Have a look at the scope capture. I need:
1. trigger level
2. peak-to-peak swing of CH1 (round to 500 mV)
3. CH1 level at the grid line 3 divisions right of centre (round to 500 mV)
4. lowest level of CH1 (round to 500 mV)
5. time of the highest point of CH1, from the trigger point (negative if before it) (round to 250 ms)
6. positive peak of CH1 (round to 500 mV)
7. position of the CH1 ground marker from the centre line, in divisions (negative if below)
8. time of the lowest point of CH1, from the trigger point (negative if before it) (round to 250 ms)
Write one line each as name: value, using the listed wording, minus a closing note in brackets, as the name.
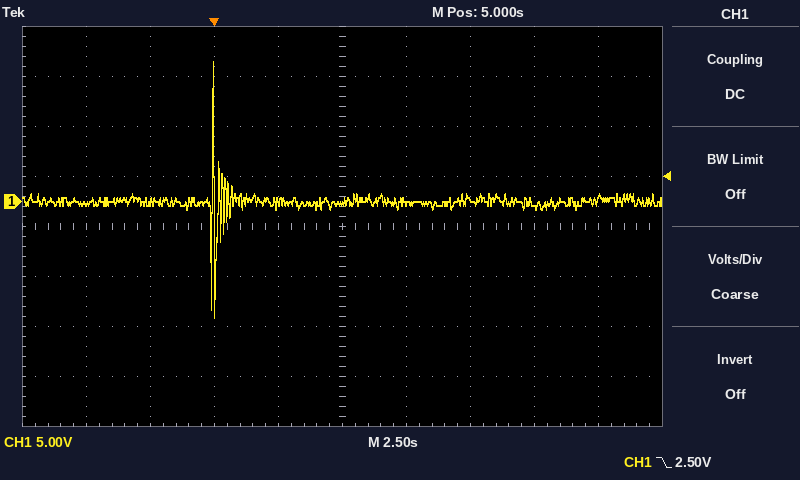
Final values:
trigger level: 2.50 V
peak-to-peak swing of CH1: 25.5 V
CH1 level at the grid line 3 divisions right of centre: -500 mV
lowest level of CH1: -11.5 V
time of the highest point of CH1, from the trigger point (negative if before it): 0.00 s
positive peak of CH1: 14.0 V
position of the CH1 ground marker from the centre line, in divisions: +0.5 div
time of the lowest point of CH1, from the trigger point (negative if before it): 0.00 s
